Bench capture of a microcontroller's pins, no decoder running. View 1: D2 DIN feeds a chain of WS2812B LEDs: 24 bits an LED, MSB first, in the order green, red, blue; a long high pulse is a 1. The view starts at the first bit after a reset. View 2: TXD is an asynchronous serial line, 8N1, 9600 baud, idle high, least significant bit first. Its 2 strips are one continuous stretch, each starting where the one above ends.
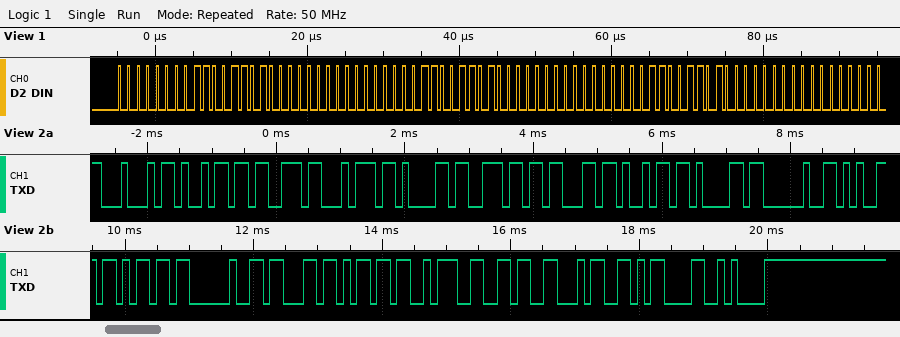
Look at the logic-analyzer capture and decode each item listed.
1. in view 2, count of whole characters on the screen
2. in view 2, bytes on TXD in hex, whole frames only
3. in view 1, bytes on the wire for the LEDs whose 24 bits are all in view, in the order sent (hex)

20
44 69 73 74 61 6E 63 69 61 20 65 6D 20 63 6D 3A 36 34 0D 0A
00 CD 00 00 CD 00 00 CD 00
